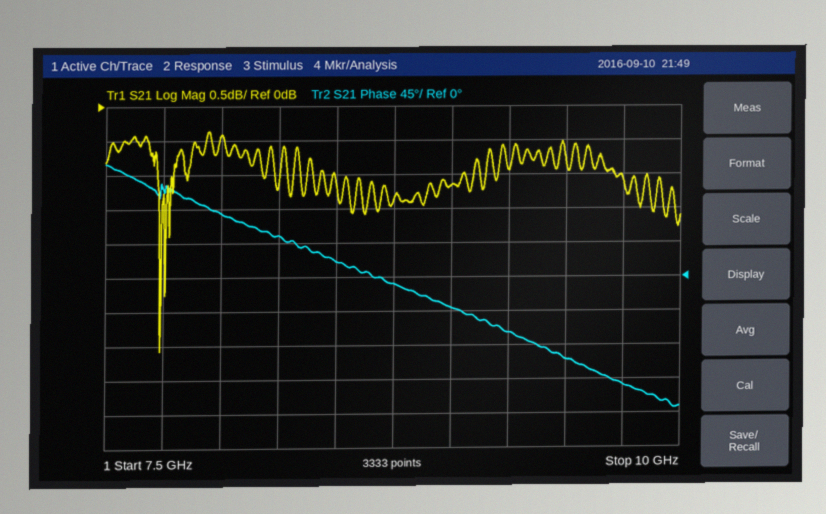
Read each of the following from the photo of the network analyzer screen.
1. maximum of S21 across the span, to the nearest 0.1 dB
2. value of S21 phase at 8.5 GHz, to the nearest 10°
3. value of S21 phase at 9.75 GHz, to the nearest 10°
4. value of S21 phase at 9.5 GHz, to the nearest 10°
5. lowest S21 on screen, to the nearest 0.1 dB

-0.4 dB
20°
-140°
-110°
-3.6 dB
